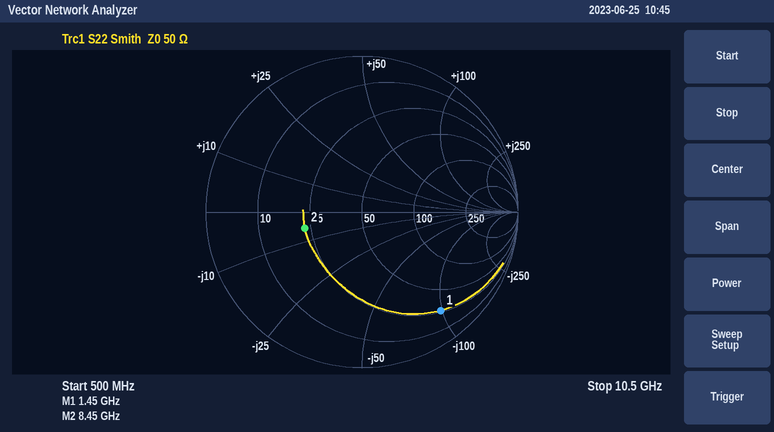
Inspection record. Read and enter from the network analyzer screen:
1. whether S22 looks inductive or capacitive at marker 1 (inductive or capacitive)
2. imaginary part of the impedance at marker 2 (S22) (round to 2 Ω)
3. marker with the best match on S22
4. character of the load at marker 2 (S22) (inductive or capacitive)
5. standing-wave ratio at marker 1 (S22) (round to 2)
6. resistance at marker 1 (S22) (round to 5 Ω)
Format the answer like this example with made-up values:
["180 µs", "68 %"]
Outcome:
["capacitive", "-6 Ω", "marker 2", "capacitive", "10", "25 Ω"]
